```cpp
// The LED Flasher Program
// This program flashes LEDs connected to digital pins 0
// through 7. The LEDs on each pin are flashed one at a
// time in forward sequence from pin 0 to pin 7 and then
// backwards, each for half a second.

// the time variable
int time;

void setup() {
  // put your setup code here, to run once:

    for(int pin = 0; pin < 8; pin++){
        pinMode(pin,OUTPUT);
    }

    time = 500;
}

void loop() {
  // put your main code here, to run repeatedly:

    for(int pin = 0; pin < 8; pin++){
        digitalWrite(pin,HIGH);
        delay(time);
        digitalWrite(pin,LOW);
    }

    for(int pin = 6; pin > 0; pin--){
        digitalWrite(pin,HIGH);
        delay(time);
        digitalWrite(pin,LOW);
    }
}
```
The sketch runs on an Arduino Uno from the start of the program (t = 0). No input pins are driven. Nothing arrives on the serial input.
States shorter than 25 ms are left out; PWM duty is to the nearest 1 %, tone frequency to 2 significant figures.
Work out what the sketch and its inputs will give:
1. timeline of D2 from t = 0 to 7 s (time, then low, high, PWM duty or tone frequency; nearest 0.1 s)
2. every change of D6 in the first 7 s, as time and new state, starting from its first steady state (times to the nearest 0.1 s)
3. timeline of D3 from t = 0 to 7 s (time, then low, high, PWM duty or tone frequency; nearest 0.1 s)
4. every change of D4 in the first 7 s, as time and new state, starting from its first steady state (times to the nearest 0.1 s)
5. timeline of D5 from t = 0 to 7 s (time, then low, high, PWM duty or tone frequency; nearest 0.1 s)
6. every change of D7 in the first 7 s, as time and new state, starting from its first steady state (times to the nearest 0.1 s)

0 s low; 1 s high; 1.5 s low; 6 s high; 6.5 s low
0 s low; 3 s high; 3.5 s low; 4 s high; 4.5 s low
0 s low; 1.5 s high; 2 s low; 5.5 s high; 6 s low
0 s low; 2 s high; 2.5 s low; 5 s high; 5.5 s low
0 s low; 2.5 s high; 3 s low; 4.5 s high; 5 s low
0 s low; 3.5 s high; 4 s low
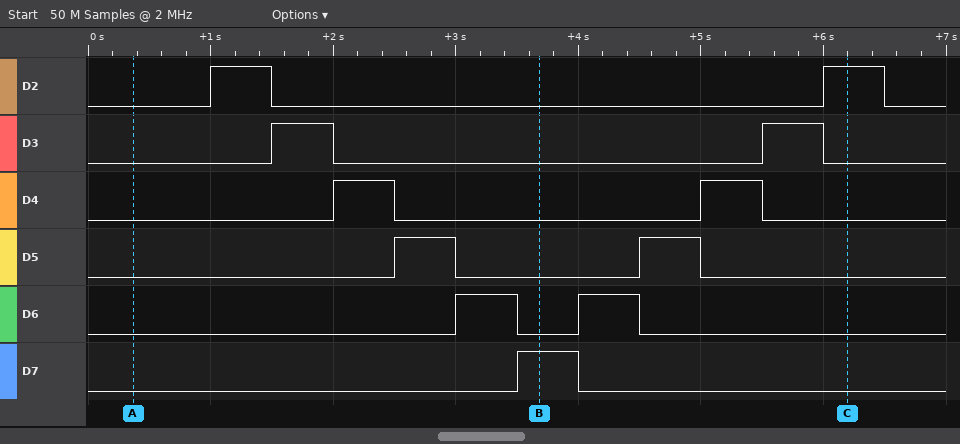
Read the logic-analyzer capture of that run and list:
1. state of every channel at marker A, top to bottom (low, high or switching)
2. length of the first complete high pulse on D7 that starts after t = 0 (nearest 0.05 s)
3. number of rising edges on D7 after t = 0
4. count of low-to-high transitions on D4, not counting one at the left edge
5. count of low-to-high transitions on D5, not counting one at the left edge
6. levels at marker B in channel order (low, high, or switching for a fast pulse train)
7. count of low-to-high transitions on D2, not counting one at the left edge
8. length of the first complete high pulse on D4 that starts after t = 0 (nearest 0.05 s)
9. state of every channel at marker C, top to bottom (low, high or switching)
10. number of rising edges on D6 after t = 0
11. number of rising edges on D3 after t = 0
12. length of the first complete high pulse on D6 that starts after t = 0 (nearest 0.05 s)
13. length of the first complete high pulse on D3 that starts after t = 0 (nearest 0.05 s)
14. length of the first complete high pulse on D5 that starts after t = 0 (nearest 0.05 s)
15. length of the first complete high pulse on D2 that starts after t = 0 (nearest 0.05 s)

D2 low, D3 low, D4 low, D5 low, D6 low, D7 low
0.50 s
1
2
2
D2 low, D3 low, D4 low, D5 low, D6 low, D7 high
2
0.50 s
D2 high, D3 low, D4 low, D5 low, D6 low, D7 low
2
2
0.50 s
0.50 s
0.50 s
0.50 s
